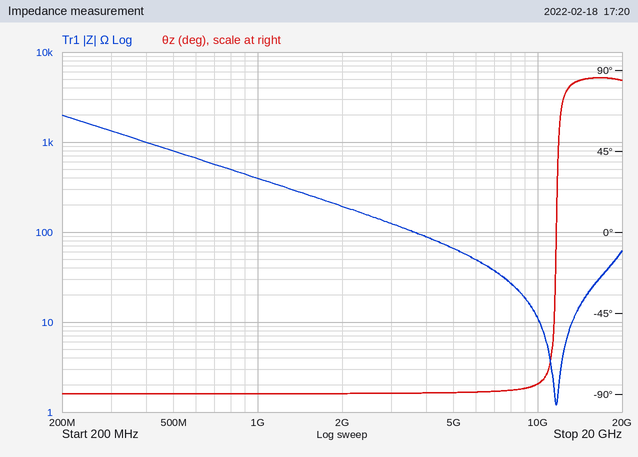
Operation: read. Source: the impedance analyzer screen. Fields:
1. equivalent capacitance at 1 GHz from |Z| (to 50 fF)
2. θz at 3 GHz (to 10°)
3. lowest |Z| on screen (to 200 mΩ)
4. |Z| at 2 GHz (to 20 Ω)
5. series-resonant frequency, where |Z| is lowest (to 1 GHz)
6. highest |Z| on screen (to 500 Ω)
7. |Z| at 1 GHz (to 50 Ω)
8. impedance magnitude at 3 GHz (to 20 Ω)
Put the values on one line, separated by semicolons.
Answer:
400 fF; -90°; 1.2 Ω; 200 Ω; 12 GHz; 2.0 kΩ; 400 Ω; 120 Ω
